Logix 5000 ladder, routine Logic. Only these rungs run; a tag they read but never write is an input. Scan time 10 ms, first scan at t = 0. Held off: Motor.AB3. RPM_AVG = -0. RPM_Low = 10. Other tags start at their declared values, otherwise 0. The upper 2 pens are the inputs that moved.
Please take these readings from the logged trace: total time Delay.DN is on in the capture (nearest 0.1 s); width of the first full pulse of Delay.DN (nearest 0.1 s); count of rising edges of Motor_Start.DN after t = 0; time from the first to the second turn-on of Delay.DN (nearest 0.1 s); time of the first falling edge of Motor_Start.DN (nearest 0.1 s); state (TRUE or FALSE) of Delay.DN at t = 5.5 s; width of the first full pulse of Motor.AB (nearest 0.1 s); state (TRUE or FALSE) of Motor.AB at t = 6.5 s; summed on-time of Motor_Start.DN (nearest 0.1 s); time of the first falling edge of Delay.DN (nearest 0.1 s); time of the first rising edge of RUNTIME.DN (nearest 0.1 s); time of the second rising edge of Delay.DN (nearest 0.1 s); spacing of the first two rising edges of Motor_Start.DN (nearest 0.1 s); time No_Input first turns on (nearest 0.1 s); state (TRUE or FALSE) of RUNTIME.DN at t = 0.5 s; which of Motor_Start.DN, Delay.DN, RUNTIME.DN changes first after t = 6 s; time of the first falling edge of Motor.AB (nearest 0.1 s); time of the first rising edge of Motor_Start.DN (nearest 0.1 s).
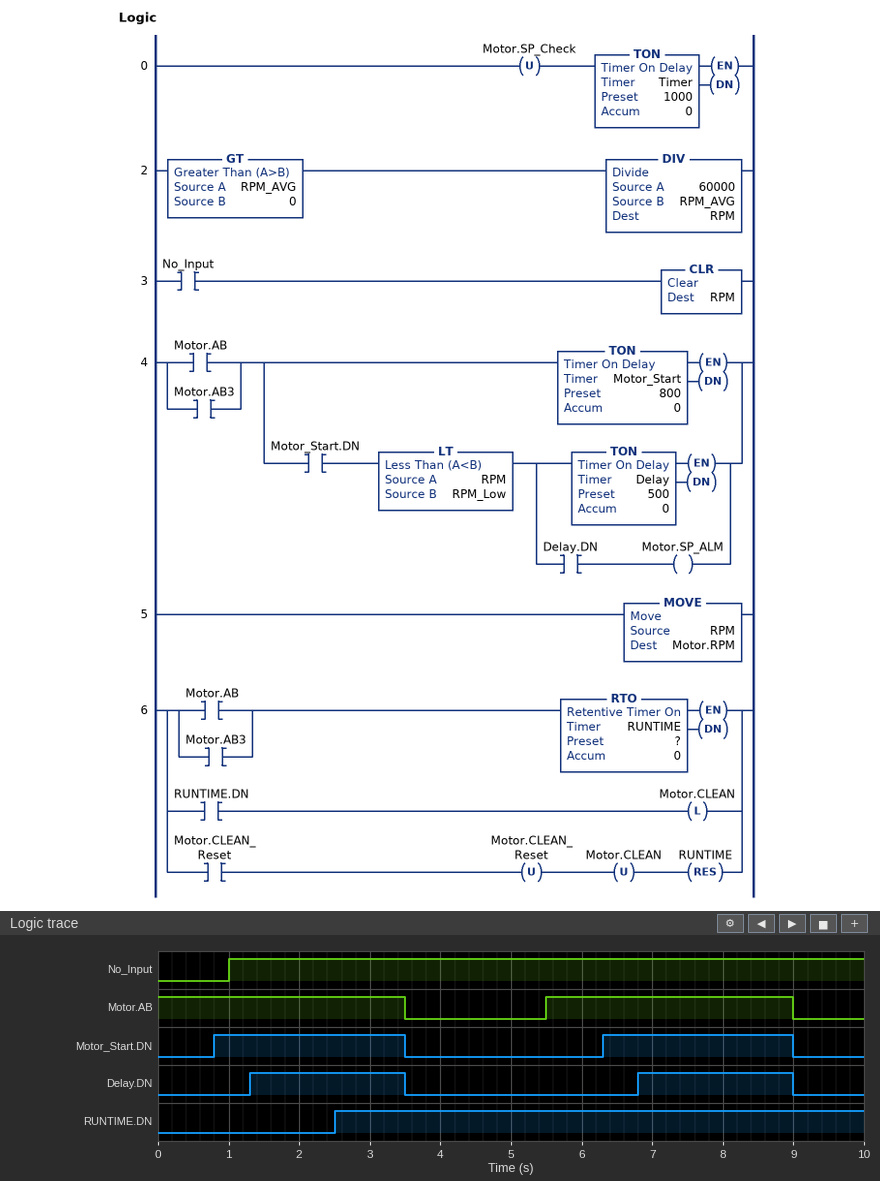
4.4 s
2.2 s
2
5.5 s
3.5 s
FALSE
3.5 s
TRUE
5.4 s
3.5 s
2.5 s
6.8 s
5.5 s
1.0 s
FALSE
Motor_Start.DN
3.5 s
0.8 s
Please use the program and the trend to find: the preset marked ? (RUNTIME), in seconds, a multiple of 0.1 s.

2.5 s
